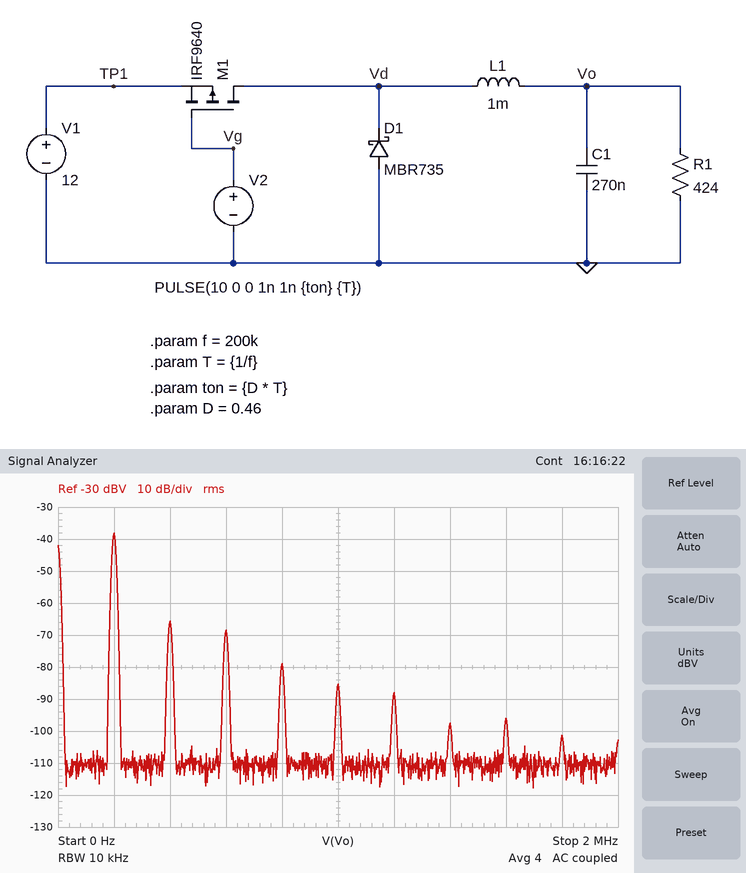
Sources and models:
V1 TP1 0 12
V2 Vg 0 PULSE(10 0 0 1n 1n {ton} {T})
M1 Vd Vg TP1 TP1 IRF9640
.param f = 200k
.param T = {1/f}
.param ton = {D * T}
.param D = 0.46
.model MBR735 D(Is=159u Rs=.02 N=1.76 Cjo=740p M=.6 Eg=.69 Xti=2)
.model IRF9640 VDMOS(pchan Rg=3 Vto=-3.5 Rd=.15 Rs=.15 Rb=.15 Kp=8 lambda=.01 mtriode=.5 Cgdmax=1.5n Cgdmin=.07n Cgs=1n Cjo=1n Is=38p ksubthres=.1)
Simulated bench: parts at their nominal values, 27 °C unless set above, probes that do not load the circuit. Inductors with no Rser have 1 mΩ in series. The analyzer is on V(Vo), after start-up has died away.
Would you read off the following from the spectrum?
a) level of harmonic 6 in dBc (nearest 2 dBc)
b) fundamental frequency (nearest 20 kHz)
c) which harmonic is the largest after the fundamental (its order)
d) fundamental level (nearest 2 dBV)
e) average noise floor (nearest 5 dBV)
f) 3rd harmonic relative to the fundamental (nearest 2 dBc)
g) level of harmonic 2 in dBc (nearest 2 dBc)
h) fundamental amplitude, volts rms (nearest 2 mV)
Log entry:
-50 dBc
200 kHz
2
-38 dBV
-110 dBV
-30 dBc
-28 dBc
12 mV
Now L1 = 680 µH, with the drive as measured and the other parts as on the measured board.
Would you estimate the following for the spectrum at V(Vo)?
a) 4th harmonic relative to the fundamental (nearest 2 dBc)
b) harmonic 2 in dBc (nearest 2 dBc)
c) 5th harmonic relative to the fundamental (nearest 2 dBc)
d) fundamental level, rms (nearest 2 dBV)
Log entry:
-42 dBc
-30 dBc
-46 dBc
-34 dBV
